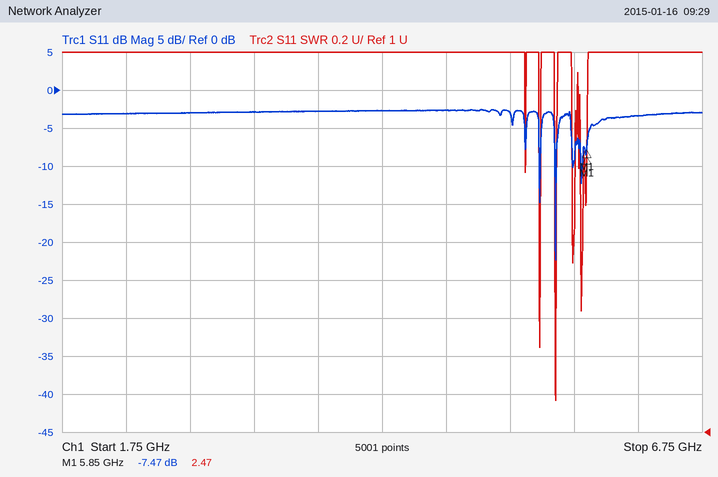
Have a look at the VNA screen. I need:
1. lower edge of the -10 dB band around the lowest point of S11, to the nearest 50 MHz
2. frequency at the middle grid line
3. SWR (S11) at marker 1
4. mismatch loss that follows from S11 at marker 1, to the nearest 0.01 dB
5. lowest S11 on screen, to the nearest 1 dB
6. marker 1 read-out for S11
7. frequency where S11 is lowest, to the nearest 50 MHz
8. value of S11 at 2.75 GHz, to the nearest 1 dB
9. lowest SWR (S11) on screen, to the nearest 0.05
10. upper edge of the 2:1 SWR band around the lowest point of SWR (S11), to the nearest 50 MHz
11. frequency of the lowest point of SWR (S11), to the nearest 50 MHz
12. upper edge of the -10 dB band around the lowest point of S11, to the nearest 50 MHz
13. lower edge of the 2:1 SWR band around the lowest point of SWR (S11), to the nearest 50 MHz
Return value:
5.60 GHz
4.25 GHz
2.47
0.86 dB
-22 dB
-7.47 dB
5.60 GHz
-3 dB
1.15
5.60 GHz
5.60 GHz
5.60 GHz
5.60 GHz
